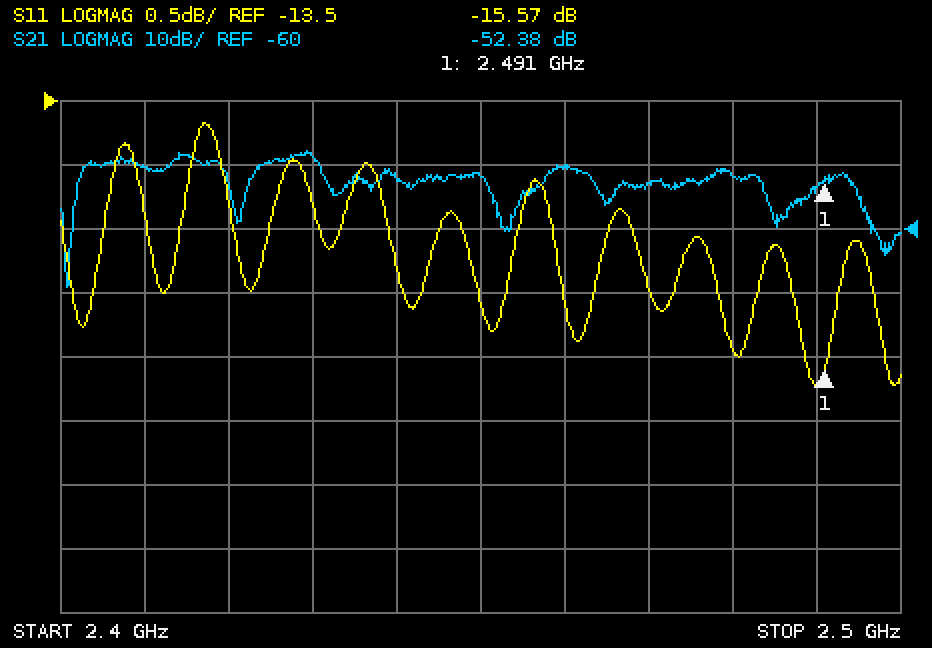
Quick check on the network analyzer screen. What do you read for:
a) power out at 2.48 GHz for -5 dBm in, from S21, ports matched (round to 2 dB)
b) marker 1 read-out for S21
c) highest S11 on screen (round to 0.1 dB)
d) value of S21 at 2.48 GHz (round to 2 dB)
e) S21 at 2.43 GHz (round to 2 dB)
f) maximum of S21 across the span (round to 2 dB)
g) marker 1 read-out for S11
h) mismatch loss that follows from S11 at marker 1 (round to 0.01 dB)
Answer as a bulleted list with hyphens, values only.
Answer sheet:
- -56 dBm
- -52.38 dB
- -13.7 dB
- -52 dB
- -48 dB
- -48 dB
- -15.57 dB
- 0.12 dB
